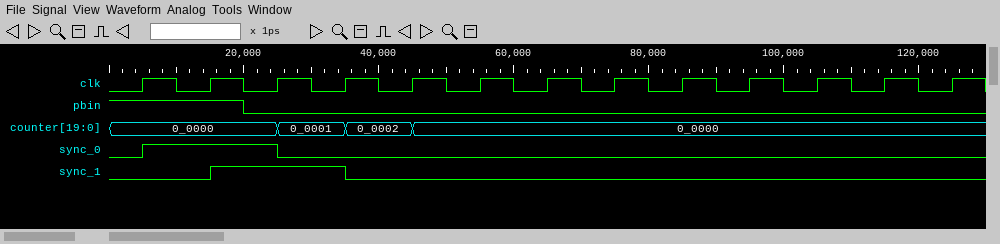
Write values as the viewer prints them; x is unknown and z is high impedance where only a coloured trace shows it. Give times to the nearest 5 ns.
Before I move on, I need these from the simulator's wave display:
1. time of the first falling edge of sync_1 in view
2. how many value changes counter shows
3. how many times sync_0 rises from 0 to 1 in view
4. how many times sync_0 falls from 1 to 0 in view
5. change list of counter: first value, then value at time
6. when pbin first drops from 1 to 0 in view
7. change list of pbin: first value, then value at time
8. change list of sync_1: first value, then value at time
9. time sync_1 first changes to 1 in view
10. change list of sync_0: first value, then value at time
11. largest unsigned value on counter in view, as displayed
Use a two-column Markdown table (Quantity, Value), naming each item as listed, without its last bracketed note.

| Quantity | Value |
|---|---|
| time of the first falling edge of sync_1 in view | 35 ns |
| how many value changes counter shows | 3 |
| how many times sync_0 rises from 0 to 1 in view | 1 |
| how many times sync_0 falls from 1 to 0 in view | 1 |
| change list of counter: first value, then value at time | 0_0000, 0_0001 at 25 ns, 0_0002 at 35 ns, 0_0000 at 45 ns |
| when pbin first drops from 1 to 0 in view | 20 ns |
| change list of pbin: first value, then value at time | 1, 0 at 20 ns |
| change list of sync_1: first value, then value at time | 0, 1 at 15 ns, 0 at 35 ns |
| time sync_1 first changes to 1 in view | 15 ns |
| change list of sync_0: first value, then value at time | 0, 1 at 5 ns, 0 at 25 ns |
| largest unsigned value on counter in view, as displayed | 0_0002 |
